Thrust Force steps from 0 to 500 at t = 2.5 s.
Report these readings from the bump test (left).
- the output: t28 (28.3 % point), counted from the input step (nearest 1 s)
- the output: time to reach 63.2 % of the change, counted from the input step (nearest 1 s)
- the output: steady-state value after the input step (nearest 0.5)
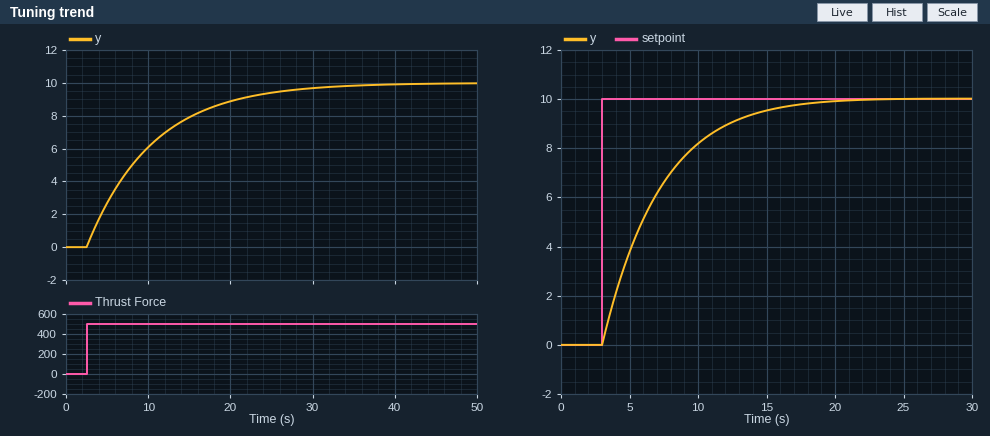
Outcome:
3 s
8 s
10.0
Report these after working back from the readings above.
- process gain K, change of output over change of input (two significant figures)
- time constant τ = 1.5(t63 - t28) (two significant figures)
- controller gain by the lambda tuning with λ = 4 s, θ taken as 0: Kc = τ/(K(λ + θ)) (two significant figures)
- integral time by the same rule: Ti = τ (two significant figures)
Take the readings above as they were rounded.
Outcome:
0.020
7.5 s
94
7.5 s
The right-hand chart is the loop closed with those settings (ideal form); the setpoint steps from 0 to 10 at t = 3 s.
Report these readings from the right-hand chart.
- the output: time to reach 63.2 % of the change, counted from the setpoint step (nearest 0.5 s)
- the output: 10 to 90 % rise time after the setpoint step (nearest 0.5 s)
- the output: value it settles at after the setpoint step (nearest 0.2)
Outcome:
4.0 s
9.0 s
10.0
